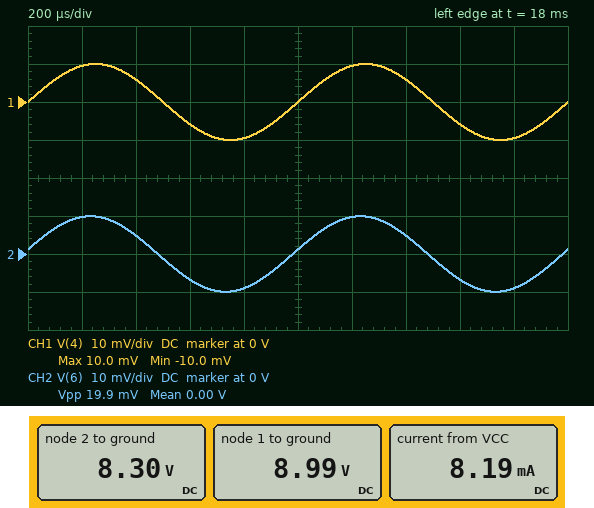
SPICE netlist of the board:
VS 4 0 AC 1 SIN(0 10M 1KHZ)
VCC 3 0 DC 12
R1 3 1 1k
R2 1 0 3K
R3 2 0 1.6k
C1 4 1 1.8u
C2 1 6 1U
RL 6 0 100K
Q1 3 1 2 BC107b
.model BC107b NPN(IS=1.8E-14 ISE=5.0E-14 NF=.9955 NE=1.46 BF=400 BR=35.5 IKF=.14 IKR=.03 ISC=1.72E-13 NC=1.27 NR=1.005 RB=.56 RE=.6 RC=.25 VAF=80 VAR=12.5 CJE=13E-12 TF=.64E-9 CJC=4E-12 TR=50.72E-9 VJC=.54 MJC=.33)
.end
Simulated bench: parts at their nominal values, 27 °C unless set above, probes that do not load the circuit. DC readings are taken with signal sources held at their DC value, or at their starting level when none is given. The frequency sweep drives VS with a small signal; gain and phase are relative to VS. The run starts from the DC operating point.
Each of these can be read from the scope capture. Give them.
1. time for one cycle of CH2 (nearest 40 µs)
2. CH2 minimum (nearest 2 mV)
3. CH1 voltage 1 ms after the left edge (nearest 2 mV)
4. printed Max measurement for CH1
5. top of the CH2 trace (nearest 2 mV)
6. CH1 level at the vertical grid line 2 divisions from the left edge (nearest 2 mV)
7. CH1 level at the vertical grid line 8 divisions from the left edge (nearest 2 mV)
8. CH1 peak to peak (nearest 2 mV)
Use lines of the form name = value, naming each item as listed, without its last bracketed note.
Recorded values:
time for one cycle of CH2 = 1.00 ms
CH2 minimum = -10 mV
CH1 voltage 1 ms after the left edge = 0 V
printed Max measurement for CH1 = 10.0 mV
top of the CH2 trace = 10 mV
CH1 level at the vertical grid line 2 divisions from the left edge = 6 mV
CH1 level at the vertical grid line 8 divisions from the left edge = -6 mV
CH1 peak to peak = 20 mV
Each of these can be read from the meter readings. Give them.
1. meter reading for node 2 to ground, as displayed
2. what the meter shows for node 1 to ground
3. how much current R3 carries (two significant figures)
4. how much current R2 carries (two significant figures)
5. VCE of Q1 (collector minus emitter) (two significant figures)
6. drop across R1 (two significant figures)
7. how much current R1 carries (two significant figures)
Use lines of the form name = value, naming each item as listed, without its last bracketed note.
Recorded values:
meter reading for node 2 to ground, as displayed = 8.30 V
what the meter shows for node 1 to ground = 8.99 V
how much current R3 carries = 5.2 mA
how much current R2 carries = 3.0 mA
VCE of Q1 (collector minus emitter) = 3.7 V
drop across R1 = 3.0 V
how much current R1 carries = 3.0 mA
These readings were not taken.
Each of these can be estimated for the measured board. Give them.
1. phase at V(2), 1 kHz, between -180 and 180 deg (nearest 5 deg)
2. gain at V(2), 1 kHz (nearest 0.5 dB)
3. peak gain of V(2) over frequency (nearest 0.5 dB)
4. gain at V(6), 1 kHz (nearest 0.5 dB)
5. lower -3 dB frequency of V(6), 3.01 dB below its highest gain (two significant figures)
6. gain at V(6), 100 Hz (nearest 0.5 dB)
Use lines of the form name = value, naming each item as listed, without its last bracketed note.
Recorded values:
phase at V(2), 1 kHz, between -180 and 180 deg = 5 deg
gain at V(2), 1 kHz = 0 dB
peak gain of V(2) over frequency = 0 dB
gain at V(6), 1 kHz = 0 dB
lower -3 dB frequency of V(6), 3.01 dB below its highest gain = 120 Hz
gain at V(6), 100 Hz = -4.0 dB
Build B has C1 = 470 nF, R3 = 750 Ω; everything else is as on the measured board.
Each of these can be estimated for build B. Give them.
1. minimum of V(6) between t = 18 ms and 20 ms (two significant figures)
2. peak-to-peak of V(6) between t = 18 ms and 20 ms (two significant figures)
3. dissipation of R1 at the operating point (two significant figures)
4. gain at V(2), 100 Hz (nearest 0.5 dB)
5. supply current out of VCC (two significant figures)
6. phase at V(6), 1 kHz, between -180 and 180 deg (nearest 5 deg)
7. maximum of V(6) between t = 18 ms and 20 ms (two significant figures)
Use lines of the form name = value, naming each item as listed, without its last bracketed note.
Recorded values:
minimum of V(6) between t = 18 ms and 20 ms = -9.1 mV
peak-to-peak of V(6) between t = 18 ms and 20 ms = 18 mV
dissipation of R1 at the operating point = 9.2 mW
gain at V(2), 100 Hz = -13.5 dB
supply current out of VCC = 14 mA
phase at V(6), 1 kHz, between -180 and 180 deg = 25 deg
maximum of V(6) between t = 18 ms and 20 ms = 9.1 mV
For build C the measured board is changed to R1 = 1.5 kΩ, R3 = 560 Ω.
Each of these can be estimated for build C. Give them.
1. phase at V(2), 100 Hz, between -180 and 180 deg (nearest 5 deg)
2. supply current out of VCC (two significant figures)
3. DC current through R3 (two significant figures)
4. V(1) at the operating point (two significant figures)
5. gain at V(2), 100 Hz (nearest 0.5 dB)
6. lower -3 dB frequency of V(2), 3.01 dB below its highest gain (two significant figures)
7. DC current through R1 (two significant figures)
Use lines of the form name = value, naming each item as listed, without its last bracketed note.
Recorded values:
phase at V(2), 100 Hz, between -180 and 180 deg = 40 deg
supply current out of VCC = 16 mA
DC current through R3 = 13 mA
V(1) at the operating point = 8.0 V
gain at V(2), 100 Hz = -2.5 dB
lower -3 dB frequency of V(2), 3.01 dB below its highest gain = 90 Hz
DC current through R1 = 2.7 mA
